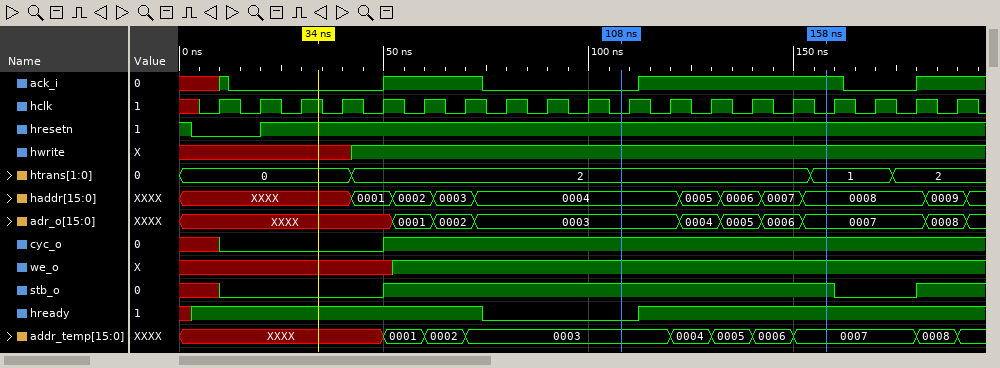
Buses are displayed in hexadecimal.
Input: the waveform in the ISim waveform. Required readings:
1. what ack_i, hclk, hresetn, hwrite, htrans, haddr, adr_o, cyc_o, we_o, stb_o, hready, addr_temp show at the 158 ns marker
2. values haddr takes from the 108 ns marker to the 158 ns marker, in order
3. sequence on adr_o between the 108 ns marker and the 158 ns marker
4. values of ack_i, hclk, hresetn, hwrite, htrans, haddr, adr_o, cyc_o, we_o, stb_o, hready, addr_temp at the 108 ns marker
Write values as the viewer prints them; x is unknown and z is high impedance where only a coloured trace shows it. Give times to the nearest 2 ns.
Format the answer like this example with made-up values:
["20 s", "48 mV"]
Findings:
["ack_i=1, hclk=0, hresetn=1, hwrite=1, htrans=1, haddr=0008, adr_o=0007, cyc_o=1, we_o=1, stb_o=1, hready=1, addr_temp=0007", "0004, 0005, 0006, 0007, 0008", "0003, 0004, 0005, 0006, 0007", "ack_i=0, hclk=0, hresetn=1, hwrite=1, htrans=2, haddr=0004, adr_o=0003, cyc_o=1, we_o=1, stb_o=1, hready=0, addr_temp=0003"]
